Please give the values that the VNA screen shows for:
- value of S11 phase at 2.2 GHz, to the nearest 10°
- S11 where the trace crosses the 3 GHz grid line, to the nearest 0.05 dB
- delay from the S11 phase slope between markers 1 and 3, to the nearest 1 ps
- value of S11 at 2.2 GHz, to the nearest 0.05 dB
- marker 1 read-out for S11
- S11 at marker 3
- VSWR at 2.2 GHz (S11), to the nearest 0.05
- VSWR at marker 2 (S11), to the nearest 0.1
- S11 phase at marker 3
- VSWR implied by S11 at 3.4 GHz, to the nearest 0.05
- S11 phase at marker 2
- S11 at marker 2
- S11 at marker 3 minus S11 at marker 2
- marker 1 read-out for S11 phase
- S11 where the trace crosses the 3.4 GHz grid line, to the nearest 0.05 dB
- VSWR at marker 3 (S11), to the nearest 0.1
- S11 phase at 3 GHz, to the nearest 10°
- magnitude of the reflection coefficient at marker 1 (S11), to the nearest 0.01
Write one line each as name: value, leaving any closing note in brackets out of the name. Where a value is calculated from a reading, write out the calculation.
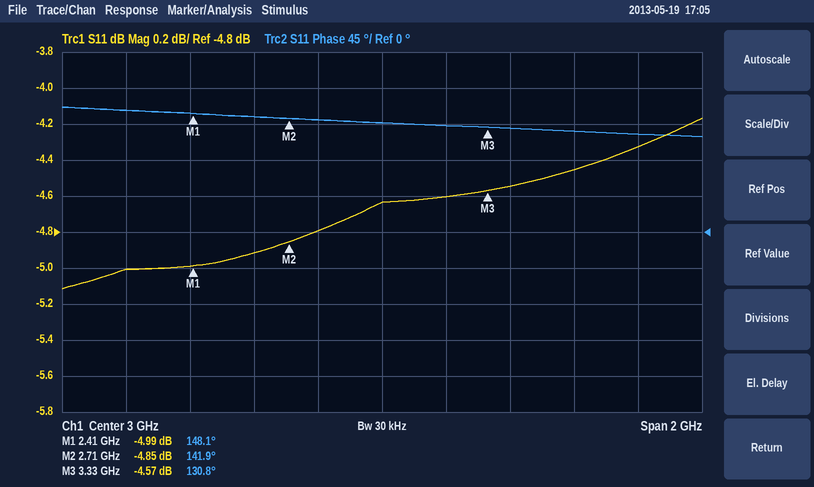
value of S11 phase at 2.2 GHz, to the nearest 10°: 150°
S11 where the trace crosses the 3 GHz grid line, to the nearest 0.05 dB: -4.65 dB
delay from the S11 phase slope between markers 1 and 3, to the nearest 1 ps: −(130.8° − (148.1°))/(360° × 920 MHz) ≈ 52 ps
value of S11 at 2.2 GHz, to the nearest 0.05 dB: -5.00 dB
marker 1 read-out for S11: -4.99 dB
S11 at marker 3: -4.57 dB
VSWR at 2.2 GHz (S11), to the nearest 0.05: |Γ| = 10^(-5/20) = 0.5623; VSWR = (1 + 0.5623)/(1 − 0.5623) ≈ 3.57, so 3.55 to the nearest 0.05
VSWR at marker 2 (S11), to the nearest 0.1: (1 + 0.5721)/(1 − 0.5721) ≈ 3.7
S11 phase at marker 3: 130.8°
VSWR implied by S11 at 3.4 GHz, to the nearest 0.05: |Γ| = 10^(-4.55/20) = 0.5922; VSWR = (1 + 0.5922)/(1 − 0.5922) ≈ 3.90
S11 phase at marker 2: 141.9°
S11 at marker 2: -4.85 dB
S11 at marker 3 minus S11 at marker 2: -4.57 − (-4.85) = 0.28 dB
marker 1 read-out for S11 phase: 148.1°
S11 where the trace crosses the 3.4 GHz grid line, to the nearest 0.05 dB: -4.55 dB
VSWR at marker 3 (S11), to the nearest 0.1: (1 + 0.5909)/(1 − 0.5909) ≈ 3.9
S11 phase at 3 GHz, to the nearest 10°: 140°
magnitude of the reflection coefficient at marker 1 (S11), to the nearest 0.01: 10^(-4.99/20) ≈ 0.56
